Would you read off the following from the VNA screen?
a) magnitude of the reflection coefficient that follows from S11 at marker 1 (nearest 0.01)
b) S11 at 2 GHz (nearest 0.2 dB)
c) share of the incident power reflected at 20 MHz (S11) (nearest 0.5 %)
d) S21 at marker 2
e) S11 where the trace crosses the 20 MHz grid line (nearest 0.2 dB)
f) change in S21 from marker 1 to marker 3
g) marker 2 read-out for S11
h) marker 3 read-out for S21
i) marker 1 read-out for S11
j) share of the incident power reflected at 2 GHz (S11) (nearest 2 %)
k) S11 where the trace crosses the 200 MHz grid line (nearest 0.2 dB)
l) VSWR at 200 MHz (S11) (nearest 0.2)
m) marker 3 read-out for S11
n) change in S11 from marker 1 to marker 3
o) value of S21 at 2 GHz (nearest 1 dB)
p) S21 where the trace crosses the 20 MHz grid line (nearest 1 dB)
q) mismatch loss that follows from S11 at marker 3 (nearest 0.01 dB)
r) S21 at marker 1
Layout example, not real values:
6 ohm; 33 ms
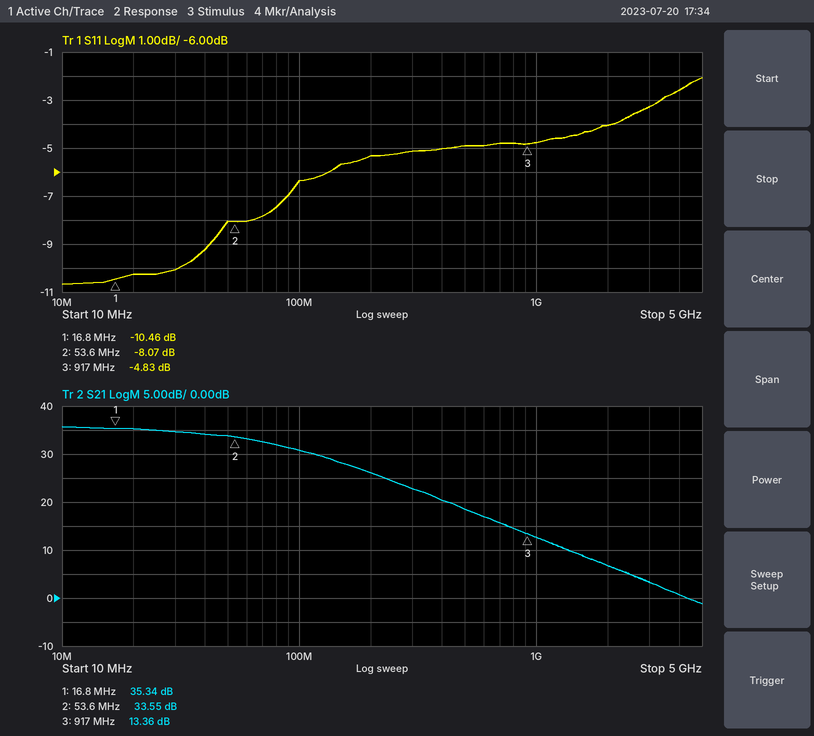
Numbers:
0.30; -4.0 dB; 9.5 %; 33.55 dB; -10.2 dB; -21.98 dB; -8.07 dB; 13.36 dB; -10.46 dB; 40 %; -5.4 dB; 3.4; -4.83 dB; 5.63 dB; 7 dB; 35 dB; 1.73 dB; 35.34 dB
